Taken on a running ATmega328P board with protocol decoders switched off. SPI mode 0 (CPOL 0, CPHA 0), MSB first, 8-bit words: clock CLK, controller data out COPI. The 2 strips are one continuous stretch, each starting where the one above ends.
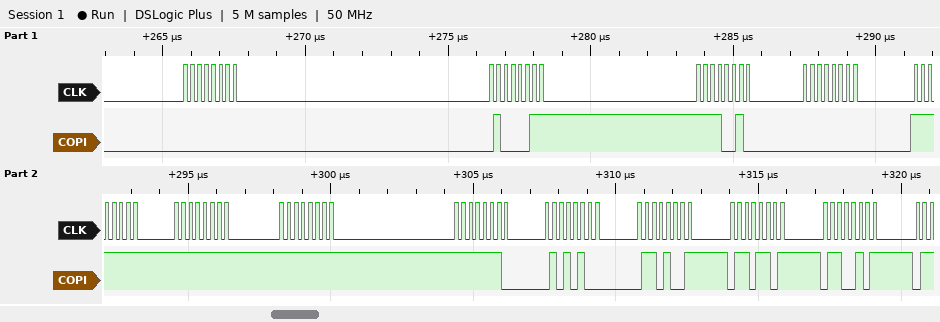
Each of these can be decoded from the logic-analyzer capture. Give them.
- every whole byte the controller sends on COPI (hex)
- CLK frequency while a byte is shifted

00 43 F2 00 FF FF FF FE 54 69 6D 65
4 MHz
